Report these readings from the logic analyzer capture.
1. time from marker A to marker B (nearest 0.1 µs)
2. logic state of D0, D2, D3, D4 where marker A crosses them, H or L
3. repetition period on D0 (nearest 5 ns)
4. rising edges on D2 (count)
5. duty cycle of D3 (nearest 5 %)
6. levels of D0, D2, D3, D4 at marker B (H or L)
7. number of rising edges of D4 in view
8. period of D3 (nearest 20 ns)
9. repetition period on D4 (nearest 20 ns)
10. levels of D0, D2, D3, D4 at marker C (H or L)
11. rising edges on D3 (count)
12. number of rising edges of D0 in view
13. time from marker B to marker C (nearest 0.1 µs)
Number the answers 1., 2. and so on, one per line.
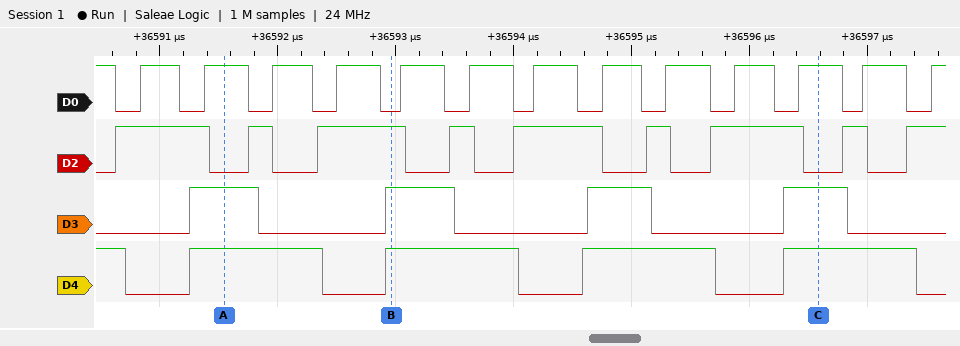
1. 1.4 µs
2. D0=H, D2=L, D3=H, D4=H
3. 560 ns
4. 9
5. 35 %
6. D0=L, D2=H, D3=H, D4=H
7. 4
8. 1680 ns
9. 1680 ns
10. D0=H, D2=L, D3=H, D4=H
11. 4
12. 13
13. 3.6 µs
